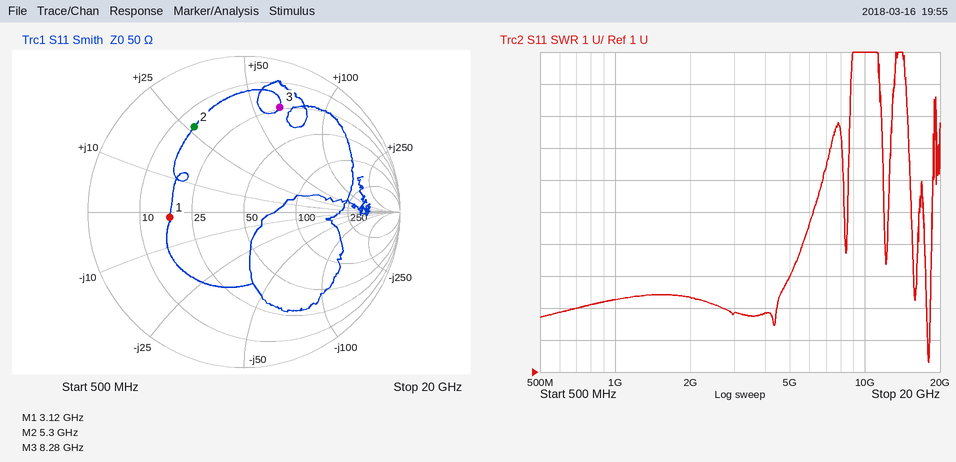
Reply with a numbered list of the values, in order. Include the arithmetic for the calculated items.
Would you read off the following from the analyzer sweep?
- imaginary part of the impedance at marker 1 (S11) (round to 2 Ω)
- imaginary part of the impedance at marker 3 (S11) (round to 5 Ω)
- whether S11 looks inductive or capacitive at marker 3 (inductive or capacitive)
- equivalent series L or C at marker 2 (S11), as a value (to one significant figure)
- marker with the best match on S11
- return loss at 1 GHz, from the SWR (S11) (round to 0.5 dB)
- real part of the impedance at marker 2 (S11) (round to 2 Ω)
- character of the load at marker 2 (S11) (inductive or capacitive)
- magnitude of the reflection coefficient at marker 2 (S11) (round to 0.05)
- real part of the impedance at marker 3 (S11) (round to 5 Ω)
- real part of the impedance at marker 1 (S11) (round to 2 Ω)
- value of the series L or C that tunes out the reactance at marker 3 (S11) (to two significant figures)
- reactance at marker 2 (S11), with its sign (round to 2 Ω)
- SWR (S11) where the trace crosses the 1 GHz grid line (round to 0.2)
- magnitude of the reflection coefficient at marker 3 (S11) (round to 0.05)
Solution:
1. -2 Ω
2. +65 Ω
3. inductive
4. L = 26 Ω/(2π × 5.3 GHz) ≈ 781 pH, so 800 pH to one significant figure
5. marker 1
6. −20 log10((3.2 − 1)/(3.2 + 1)) ≈ 5.62 dB, so 5.5 dB to the nearest 0.5 dB
7. 14 Ω
8. inductive
9. 0.65
10. 25 Ω
11. 18 Ω
12. C = 1/(2π × 8.28 GHz × 65 Ω) ≈ 296 fF, so 300 fF to two significant figures
13. +26 Ω
14. 3.2
15. 0.70
